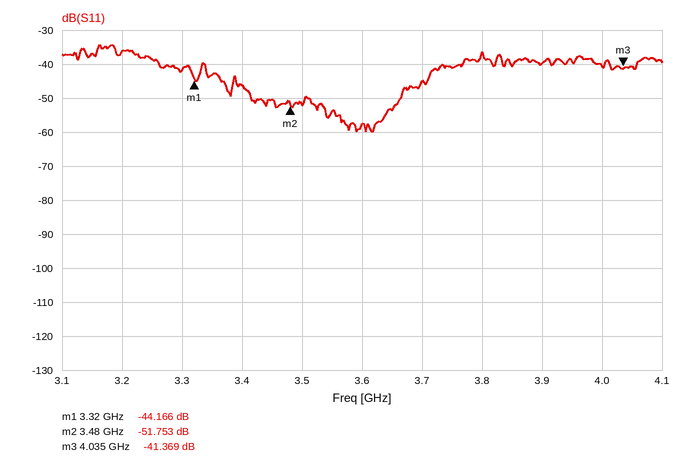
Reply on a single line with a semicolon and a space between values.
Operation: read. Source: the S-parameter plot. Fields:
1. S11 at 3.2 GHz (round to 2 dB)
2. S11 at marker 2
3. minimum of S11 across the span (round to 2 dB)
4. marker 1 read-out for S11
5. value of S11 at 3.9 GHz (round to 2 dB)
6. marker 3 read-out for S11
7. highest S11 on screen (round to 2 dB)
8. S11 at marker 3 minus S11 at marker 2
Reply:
-36 dB; -51.753 dB; -60 dB; -44.166 dB; -40 dB; -41.369 dB; -34 dB; 10.384 dB
